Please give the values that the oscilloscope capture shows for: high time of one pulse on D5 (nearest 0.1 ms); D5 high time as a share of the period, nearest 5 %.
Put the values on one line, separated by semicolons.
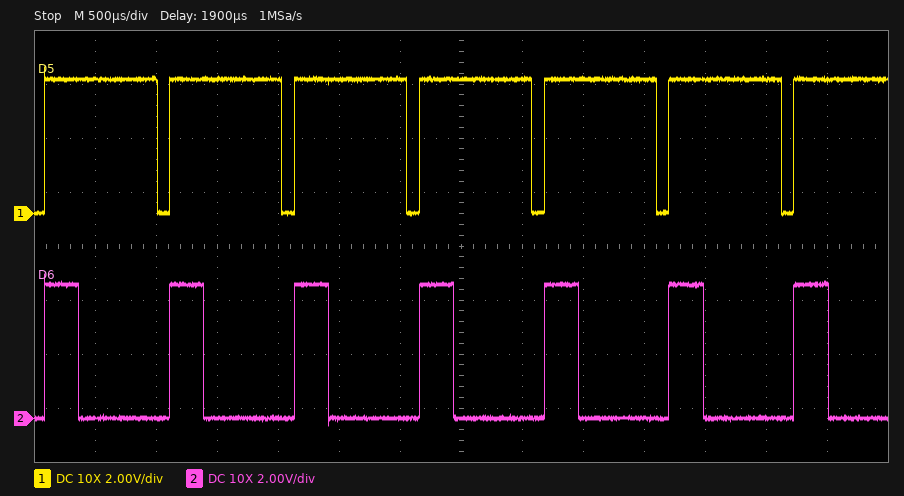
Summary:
0.9 ms; 90 %
